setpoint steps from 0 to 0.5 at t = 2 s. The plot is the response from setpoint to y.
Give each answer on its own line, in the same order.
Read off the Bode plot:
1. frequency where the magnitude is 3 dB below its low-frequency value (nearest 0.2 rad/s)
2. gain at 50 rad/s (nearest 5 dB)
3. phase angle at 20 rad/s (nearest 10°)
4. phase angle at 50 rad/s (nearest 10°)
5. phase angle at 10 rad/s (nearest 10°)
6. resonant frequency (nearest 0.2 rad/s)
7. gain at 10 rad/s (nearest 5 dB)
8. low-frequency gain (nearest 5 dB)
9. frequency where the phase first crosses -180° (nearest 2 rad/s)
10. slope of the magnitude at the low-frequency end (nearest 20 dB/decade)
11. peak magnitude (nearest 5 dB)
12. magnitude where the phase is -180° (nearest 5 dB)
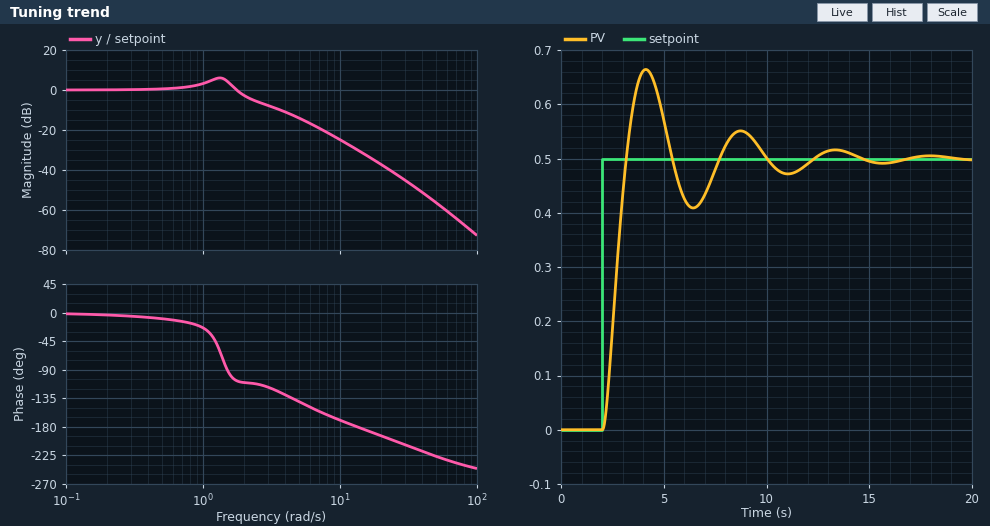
2.0 rad/s
-55 dB
-190°
-230°
-170°
1.4 rad/s
-25 dB
0 dB
14 rad/s
0 dB/decade
5 dB
-30 dB
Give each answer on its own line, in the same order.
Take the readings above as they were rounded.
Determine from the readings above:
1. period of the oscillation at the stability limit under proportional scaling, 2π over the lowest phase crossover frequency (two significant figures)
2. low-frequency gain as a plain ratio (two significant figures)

0.45 s
1.0
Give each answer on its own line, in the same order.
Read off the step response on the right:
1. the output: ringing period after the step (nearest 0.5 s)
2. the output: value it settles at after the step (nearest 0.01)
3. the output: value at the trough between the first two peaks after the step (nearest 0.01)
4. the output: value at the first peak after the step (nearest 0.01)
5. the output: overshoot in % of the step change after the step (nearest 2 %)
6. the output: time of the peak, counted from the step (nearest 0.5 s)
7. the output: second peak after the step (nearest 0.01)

4.5 s
0.50
0.41
0.66
32 %
2.0 s
0.55
